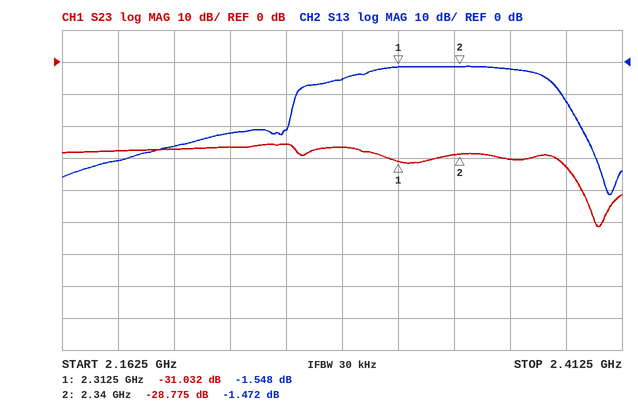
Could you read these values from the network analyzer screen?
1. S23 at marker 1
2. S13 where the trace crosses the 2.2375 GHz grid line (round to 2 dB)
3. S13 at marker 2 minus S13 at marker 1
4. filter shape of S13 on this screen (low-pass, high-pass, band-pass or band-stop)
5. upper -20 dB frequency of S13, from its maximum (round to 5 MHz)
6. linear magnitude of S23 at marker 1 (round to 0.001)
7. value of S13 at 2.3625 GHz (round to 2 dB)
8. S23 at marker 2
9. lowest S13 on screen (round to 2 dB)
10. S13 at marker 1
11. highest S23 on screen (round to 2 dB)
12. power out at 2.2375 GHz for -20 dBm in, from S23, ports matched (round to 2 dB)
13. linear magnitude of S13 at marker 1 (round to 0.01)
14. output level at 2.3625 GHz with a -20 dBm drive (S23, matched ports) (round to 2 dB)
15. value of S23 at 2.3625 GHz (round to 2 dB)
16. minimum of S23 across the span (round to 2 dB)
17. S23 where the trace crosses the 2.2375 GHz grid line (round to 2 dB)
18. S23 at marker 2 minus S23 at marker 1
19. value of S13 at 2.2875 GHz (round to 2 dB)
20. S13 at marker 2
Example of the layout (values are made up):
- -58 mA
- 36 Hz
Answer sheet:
- -31.032 dB
- -22 dB
- 0.076 dB
- band-pass
- 2.395 GHz
- 0.028
- -2 dB
- -28.775 dB
- -42 dB
- -1.548 dB
- -26 dB
- -46 dBm
- 0.84
- -50 dBm
- -30 dB
- -52 dB
- -26 dB
- 2.257 dB
- -6 dB
- -1.472 dB
